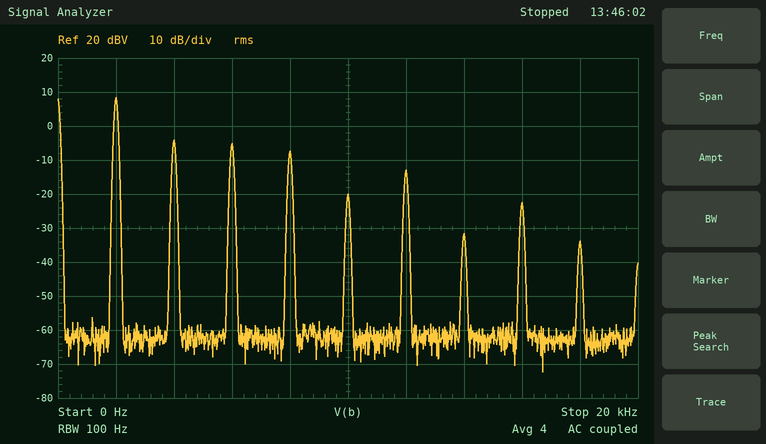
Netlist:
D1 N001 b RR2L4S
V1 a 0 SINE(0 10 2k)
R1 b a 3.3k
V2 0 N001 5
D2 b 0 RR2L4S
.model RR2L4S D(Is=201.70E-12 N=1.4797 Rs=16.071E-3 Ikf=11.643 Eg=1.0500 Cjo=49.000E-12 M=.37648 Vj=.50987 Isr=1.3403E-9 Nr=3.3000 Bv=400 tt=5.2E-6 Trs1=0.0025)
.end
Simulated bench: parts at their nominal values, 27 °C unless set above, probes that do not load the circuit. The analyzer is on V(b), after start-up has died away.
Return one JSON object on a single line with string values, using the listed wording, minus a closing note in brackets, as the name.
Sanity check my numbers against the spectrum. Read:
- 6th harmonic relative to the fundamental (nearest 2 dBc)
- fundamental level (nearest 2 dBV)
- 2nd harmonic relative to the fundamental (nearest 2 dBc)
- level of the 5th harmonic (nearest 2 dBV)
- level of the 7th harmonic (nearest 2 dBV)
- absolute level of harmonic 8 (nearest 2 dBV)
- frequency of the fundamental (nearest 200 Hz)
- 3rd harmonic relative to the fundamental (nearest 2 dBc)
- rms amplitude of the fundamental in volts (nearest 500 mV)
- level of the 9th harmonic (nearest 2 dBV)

{"6th harmonic relative to the fundamental": "-22 dBc", "fundamental level": "8 dBV", "2nd harmonic relative to the fundamental": "-12 dBc", "level of the 5th harmonic": "-20 dBV", "level of the 7th harmonic": "-32 dBV", "absolute level of harmonic 8": "-22 dBV", "frequency of the fundamental": "2.0 kHz", "3rd harmonic relative to the fundamental": "-14 dBc", "rms amplitude of the fundamental in volts": "2.5 V", "level of the 9th harmonic": "-34 dBV"}
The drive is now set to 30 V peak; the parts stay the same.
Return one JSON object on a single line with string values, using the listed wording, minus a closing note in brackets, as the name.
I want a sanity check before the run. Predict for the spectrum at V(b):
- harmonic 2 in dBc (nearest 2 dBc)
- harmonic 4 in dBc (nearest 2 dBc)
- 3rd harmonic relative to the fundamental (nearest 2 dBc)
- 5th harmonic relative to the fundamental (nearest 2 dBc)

{"harmonic 2 in dBc": "-22 dBc", "harmonic 4 in dBc": "-22 dBc", "3rd harmonic relative to the fundamental": "-10 dBc", "5th harmonic relative to the fundamental": "-16 dBc"}
